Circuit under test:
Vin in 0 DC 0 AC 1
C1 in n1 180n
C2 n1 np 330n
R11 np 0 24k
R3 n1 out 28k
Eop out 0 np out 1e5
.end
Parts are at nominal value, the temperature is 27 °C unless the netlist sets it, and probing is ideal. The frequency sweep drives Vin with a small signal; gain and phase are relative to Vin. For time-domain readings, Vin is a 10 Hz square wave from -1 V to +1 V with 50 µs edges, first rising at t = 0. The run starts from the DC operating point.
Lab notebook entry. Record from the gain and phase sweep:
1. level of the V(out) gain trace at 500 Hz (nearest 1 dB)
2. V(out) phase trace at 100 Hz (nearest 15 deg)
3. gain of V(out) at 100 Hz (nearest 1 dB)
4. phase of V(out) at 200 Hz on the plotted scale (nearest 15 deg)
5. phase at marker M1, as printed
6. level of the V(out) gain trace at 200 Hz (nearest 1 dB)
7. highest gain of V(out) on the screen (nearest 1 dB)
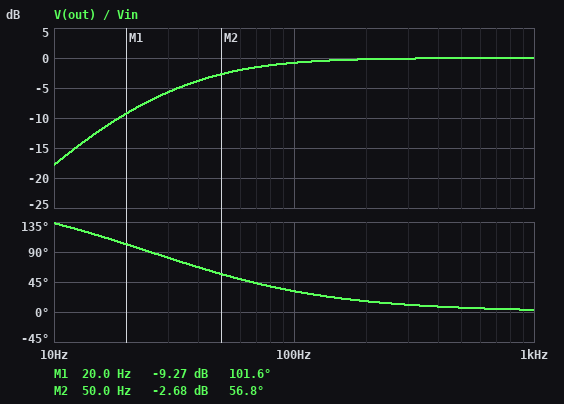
0 dB
30 deg
-1 dB
15 deg
101.6 deg
0 dB
0 dB
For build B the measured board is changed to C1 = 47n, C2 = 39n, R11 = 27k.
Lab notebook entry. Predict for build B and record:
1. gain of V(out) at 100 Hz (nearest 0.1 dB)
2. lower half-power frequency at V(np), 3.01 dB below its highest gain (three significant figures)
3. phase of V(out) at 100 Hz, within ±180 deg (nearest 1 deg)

-9.2 dB
217 Hz
107 deg
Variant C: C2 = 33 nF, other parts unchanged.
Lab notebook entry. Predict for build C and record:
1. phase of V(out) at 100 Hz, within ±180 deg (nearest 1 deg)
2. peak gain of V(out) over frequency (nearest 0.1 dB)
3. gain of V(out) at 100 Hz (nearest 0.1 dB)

81 deg
0 dB
-7.6 dB
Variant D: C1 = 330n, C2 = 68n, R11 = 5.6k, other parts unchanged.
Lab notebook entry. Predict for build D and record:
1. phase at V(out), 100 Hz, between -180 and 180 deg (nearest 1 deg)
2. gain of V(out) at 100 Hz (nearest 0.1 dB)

87 deg
-14.1 dB
